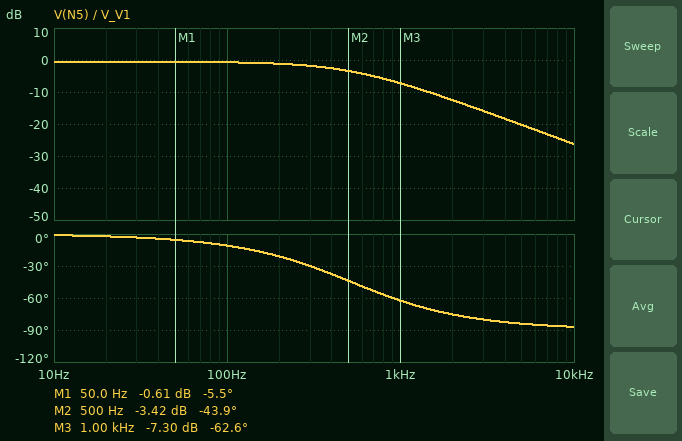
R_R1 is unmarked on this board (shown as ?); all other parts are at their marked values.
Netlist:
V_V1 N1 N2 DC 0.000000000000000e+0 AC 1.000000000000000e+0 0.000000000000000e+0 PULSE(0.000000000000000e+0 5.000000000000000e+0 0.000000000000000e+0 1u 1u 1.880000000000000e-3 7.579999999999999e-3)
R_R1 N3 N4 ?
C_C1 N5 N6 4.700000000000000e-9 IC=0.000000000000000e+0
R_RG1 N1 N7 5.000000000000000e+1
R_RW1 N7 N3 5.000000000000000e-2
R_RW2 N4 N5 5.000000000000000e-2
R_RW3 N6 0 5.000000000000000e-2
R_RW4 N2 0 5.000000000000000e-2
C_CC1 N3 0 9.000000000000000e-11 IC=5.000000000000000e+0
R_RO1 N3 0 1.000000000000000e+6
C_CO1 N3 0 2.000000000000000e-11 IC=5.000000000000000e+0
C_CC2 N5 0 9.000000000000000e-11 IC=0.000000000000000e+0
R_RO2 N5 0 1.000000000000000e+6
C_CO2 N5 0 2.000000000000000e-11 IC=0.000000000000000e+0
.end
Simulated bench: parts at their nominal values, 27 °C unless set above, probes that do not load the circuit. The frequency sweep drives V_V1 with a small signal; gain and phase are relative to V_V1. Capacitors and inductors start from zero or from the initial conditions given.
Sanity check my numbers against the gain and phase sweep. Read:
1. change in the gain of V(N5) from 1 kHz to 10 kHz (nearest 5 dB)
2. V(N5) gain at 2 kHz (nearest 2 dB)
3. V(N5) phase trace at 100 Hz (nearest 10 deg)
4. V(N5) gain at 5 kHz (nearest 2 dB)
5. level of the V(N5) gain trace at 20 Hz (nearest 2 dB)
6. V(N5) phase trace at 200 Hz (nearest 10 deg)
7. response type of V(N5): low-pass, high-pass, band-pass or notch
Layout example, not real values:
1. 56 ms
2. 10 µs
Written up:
1. -20 dB
2. -12 dB
3. -10 deg
4. -20 dB
5. 0 dB
6. -20 deg
7. low-pass
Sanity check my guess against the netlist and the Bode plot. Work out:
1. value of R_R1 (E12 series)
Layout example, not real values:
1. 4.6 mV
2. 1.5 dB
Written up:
1. 68 kΩ
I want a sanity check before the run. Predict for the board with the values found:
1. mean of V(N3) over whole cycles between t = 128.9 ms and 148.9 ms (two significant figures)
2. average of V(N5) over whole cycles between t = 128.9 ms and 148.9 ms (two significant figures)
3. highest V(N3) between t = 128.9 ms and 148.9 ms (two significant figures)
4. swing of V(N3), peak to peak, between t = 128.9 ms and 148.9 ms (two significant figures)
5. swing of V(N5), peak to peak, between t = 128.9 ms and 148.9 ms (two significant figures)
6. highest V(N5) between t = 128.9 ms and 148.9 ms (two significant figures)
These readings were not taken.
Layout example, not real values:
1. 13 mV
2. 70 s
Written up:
1. 1.2 V
2. 1.2 V
3. 5.0 V
4. 5.0 V
5. 4.7 V
6. 4.7 V
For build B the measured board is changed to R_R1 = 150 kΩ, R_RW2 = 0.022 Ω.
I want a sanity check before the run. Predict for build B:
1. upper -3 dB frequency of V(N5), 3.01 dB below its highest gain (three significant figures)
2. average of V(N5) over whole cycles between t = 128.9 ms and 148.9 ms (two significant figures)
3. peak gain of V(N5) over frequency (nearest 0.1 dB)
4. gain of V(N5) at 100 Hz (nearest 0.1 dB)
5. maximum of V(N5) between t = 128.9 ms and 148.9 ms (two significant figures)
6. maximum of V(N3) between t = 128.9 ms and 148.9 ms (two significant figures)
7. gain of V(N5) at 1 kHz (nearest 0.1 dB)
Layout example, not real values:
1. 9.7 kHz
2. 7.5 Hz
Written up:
1. 254 Hz
2. 1.1 V
3. -1.2 dB
4. -1.8 dB
5. 4.1 V
6. 5.0 V
7. -13.4 dB
